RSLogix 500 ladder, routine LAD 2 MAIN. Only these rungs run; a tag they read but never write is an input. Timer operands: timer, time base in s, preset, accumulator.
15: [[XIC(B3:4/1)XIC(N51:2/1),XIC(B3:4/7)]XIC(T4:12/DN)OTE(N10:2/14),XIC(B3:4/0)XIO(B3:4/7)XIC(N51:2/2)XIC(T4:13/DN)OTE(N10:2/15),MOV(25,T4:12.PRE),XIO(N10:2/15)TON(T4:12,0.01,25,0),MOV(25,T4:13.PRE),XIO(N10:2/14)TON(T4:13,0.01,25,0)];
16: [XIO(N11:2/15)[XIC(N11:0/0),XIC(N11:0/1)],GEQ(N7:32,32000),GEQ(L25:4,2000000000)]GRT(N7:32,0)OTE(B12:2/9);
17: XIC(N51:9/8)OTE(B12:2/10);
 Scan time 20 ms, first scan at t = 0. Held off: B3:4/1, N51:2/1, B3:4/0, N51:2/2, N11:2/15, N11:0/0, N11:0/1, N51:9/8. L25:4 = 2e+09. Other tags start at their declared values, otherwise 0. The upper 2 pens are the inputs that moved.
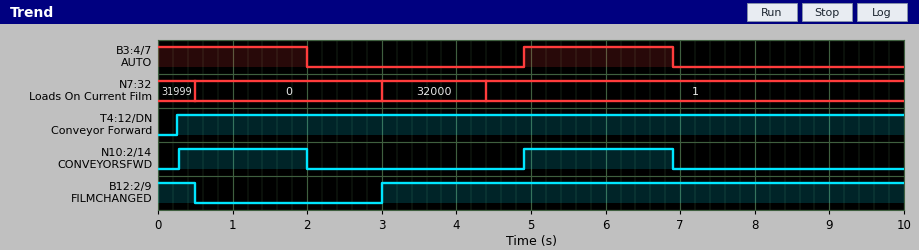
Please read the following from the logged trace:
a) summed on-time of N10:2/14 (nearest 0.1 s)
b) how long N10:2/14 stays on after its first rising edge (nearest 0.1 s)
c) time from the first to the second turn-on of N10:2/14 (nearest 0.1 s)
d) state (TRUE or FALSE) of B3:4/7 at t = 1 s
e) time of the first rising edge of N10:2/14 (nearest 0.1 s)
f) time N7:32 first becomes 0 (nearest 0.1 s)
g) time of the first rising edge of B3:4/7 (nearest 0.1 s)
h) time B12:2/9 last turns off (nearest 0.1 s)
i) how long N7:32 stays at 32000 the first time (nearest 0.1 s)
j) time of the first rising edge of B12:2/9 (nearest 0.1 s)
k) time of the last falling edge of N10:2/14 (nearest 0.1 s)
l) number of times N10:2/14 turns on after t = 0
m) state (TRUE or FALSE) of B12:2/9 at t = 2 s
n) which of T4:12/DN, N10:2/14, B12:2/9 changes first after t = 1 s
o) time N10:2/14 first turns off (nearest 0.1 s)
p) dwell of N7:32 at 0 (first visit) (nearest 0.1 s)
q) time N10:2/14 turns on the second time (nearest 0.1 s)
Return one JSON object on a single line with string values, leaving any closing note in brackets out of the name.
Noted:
{"summed on-time of N10:2/14": "3.7 s", "how long N10:2/14 stays on after its first rising edge": "1.7 s", "time from the first to the second turn-on of N10:2/14": "4.6 s", "state (TRUE or FALSE) of B3:4/7 at t = 1 s": "TRUE", "time of the first rising edge of N10:2/14": "0.3 s", "time N7:32 first becomes 0": "0.5 s", "time of the first rising edge of B3:4/7": "4.9 s", "time B12:2/9 last turns off": "0.5 s", "how long N7:32 stays at 32000 the first time": "1.4 s", "time of the first rising edge of B12:2/9": "3.0 s", "time of the last falling edge of N10:2/14": "6.9 s", "number of times N10:2/14 turns on after t = 0": "2", "state (TRUE or FALSE) of B12:2/9 at t = 2 s": "FALSE", "which of T4:12/DN, N10:2/14, B12:2/9 changes first after t = 1 s": "N10:2/14", "time N10:2/14 first turns off": "2.0 s", "dwell of N7:32 at 0 (first visit)": "2.5 s", "time N10:2/14 turns on the second time": "4.9 s"}
